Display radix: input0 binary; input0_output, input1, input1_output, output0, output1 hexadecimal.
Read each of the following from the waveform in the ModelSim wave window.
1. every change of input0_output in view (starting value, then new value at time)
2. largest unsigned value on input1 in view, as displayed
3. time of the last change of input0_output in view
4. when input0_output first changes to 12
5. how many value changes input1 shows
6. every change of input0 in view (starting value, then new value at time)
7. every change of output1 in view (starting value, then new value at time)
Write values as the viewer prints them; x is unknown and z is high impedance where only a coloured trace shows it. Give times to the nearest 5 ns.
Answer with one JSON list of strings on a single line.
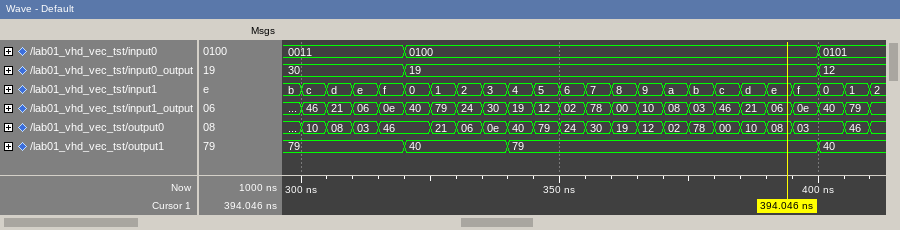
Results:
["30, 19 at 320 ns, 12 at 400 ns", "f", "400 ns", "400 ns", "23", "0011, 0100 at 320 ns, 0101 at 400 ns", "79, 40 at 320 ns, 79 at 340 ns, 40 at 400 ns"]
